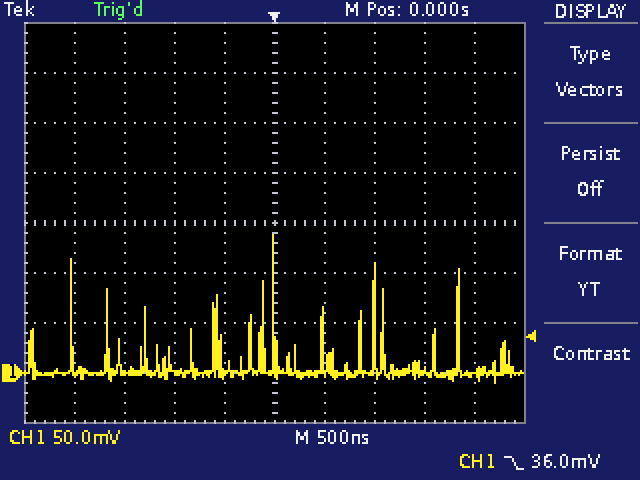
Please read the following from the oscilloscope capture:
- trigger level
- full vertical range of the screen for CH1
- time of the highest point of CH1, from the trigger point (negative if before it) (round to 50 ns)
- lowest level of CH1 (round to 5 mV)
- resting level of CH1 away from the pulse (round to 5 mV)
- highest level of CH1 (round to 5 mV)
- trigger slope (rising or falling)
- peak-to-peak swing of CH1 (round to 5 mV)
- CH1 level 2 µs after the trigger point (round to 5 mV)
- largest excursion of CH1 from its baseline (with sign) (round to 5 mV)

36.0 mV
400 mV
0 ns
-10 mV
0 mV
140 mV
falling
150 mV
0 mV
+140 mV
